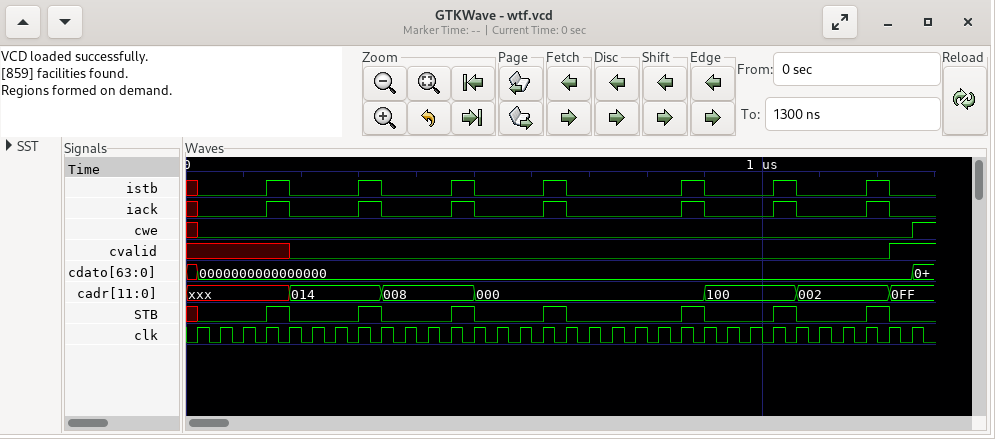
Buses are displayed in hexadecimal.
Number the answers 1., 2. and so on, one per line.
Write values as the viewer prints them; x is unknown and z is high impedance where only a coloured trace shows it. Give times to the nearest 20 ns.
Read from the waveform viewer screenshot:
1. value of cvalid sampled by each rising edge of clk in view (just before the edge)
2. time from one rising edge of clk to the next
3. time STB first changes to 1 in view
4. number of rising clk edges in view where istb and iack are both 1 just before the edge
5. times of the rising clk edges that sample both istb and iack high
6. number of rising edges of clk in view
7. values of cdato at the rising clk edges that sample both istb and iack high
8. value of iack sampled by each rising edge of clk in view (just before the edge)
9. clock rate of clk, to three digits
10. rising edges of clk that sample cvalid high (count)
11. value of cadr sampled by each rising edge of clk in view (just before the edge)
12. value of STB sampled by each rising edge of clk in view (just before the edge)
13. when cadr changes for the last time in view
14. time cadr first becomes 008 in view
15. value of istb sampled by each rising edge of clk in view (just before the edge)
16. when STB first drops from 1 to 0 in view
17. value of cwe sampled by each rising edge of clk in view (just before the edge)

1. x x x x x 0 0 0 0 0 0 0 0 0 0 0 0 0 0 0 0 0 0 0 0 0 0 0 0 0 0 1
2. 40 ns
3. 140 ns
4. 7
5. 180 ns, 340 ns, 500 ns, 660 ns, 900 ns, 1060 ns, 1220 ns
6. 32
7. 0000000000000000, 0000000000000000, 0000000000000000, 0000000000000000, 0000000000000000, 0000000000000000, 0000000000000000
8. x 0 0 0 1 0 0 0 1 0 0 0 1 0 0 0 1 0 0 0 0 0 1 0 0 0 1 0 0 0 1 0
9. 25.0 MHz
10. 1
11. xxx, xxx, xxx, xxx, xxx, 014, 014, 014, 014, 008, 008, 008, 008, 000, 000, 000, 000, 000, 000, 000, 000, 000, 000, 100, 100, 100, 100, 002, 002, 002, 002, 0FF
12. x 0 0 0 1 0 0 0 1 0 0 0 1 0 0 0 1 0 0 0 0 0 1 0 0 0 1 0 0 0 1 0
13. 1220 ns
14. 340 ns
15. x 0 0 0 1 0 0 0 1 0 0 0 1 0 0 0 1 0 0 0 0 0 1 0 0 0 1 0 0 0 1 0
16. 180 ns
17. x 0 0 0 0 0 0 0 0 0 0 0 0 0 0 0 0 0 0 0 0 0 0 0 0 0 0 0 0 0 0 0
